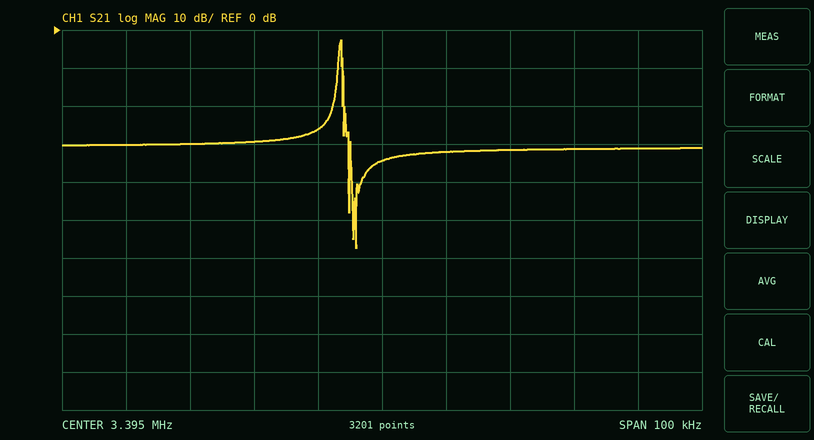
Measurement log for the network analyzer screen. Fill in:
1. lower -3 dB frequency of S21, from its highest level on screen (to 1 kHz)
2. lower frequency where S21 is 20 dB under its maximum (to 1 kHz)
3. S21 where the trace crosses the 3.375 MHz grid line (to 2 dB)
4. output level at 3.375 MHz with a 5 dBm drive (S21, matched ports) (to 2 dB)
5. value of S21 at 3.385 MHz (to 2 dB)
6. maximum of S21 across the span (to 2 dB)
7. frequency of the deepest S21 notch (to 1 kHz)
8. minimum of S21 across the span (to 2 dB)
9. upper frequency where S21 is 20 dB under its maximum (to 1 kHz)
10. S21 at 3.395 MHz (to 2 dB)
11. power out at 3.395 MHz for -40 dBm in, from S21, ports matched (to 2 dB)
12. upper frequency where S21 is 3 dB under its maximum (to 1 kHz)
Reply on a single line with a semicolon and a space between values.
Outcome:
3.388 MHz; 3.387 MHz; -30 dB; -24 dBm; -26 dB; -2 dB; 3.391 MHz; -58 dB; 3.389 MHz; -34 dB; -74 dBm; 3.389 MHz
